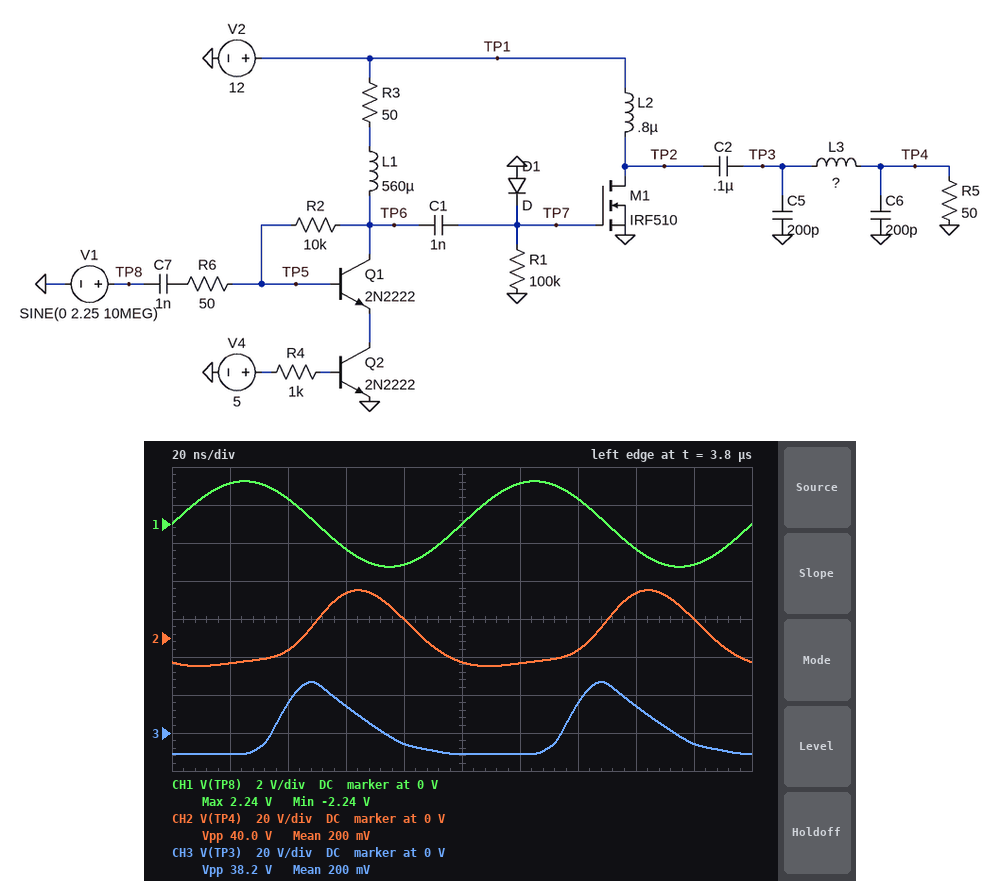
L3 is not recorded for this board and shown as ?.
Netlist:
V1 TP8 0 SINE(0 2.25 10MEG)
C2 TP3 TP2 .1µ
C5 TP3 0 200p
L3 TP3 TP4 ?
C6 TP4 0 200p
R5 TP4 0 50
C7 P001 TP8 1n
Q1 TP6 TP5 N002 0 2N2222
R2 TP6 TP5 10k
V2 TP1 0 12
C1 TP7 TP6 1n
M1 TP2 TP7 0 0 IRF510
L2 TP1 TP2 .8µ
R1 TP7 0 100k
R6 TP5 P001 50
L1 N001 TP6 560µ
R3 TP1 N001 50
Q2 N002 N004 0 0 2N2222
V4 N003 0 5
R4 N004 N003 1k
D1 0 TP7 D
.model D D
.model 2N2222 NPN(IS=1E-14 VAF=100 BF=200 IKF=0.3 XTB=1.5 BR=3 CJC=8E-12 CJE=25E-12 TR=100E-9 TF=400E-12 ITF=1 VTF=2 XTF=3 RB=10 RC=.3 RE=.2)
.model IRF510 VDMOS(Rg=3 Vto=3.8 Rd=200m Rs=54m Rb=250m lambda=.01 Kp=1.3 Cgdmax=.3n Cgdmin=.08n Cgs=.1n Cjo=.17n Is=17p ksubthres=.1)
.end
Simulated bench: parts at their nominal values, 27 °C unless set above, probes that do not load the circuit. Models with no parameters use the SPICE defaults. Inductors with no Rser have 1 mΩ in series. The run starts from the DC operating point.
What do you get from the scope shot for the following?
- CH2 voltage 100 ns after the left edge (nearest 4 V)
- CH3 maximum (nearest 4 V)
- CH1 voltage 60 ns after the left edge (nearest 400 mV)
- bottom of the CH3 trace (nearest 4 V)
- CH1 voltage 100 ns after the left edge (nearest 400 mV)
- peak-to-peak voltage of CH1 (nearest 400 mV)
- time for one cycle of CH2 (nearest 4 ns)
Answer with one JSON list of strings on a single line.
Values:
["-12 V", "28 V", "-1.2 V", "-12 V", "0 V", "4.4 V", "100 ns"]
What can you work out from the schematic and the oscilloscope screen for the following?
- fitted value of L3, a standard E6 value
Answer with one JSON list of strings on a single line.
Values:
["470 nH"]
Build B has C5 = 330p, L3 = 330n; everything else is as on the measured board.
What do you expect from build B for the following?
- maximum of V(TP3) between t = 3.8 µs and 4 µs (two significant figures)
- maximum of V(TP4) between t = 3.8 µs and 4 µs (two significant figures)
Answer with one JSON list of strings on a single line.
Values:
["26 V", "29 V"]
